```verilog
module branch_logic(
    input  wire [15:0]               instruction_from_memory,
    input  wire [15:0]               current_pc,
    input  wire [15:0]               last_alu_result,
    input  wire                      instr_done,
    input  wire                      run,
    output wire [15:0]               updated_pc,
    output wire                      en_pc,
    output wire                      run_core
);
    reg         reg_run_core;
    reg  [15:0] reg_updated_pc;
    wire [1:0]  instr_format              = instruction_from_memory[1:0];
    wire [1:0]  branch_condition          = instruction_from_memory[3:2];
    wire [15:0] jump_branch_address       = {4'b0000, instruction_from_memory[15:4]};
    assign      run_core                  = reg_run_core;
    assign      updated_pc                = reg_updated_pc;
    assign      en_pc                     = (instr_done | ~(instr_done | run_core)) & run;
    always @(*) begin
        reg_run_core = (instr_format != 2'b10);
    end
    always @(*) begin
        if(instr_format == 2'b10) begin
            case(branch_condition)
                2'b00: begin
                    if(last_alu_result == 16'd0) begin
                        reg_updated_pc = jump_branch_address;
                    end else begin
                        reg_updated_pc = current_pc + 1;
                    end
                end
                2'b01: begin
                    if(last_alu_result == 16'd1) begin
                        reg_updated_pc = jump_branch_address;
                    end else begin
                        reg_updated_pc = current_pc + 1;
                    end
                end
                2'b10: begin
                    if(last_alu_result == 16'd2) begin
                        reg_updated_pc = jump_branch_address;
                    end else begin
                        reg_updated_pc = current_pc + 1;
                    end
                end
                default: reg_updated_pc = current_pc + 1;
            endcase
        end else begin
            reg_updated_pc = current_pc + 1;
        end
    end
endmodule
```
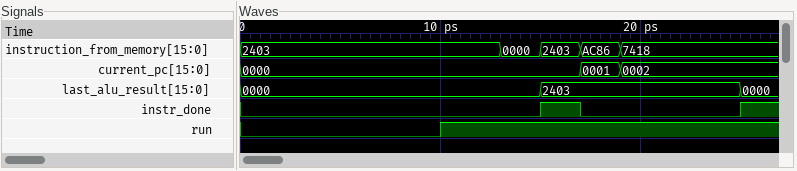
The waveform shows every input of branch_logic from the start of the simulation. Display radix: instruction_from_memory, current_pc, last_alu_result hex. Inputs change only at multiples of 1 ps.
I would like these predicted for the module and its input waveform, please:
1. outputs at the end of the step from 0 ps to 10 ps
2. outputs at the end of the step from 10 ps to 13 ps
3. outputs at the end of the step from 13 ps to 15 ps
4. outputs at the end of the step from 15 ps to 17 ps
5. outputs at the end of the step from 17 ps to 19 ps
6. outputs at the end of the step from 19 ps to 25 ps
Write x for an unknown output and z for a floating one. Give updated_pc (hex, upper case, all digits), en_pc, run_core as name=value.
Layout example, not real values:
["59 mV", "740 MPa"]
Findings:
["updated_pc=0001, en_pc=0, run_core=1", "updated_pc=0001, en_pc=0, run_core=1", "updated_pc=0001, en_pc=0, run_core=1", "updated_pc=0001, en_pc=1, run_core=1", "updated_pc=0002, en_pc=1, run_core=0", "updated_pc=0003, en_pc=0, run_core=1"]
